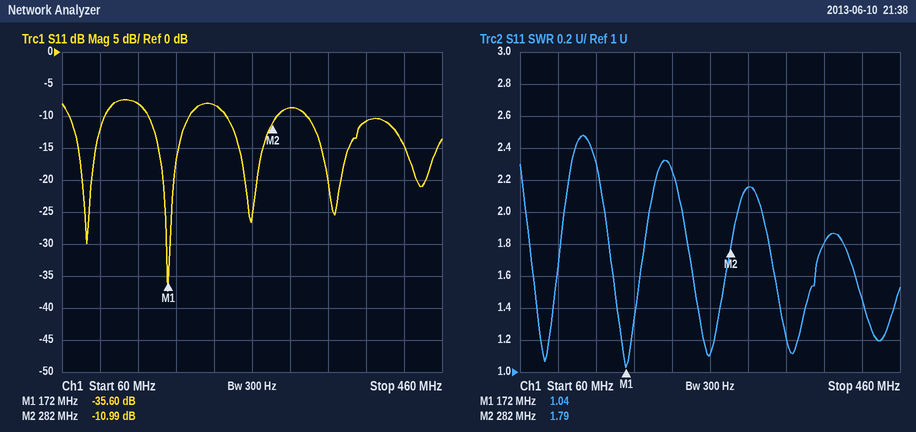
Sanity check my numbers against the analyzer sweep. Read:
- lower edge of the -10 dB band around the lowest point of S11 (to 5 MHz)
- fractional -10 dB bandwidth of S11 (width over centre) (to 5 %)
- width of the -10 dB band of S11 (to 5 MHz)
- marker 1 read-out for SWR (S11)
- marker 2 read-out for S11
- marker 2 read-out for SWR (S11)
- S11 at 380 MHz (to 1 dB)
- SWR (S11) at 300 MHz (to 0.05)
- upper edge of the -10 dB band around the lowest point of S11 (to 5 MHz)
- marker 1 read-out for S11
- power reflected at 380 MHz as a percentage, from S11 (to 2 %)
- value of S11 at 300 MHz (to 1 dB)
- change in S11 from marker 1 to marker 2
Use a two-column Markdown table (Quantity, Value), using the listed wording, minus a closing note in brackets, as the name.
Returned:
| Quantity | Value |
|---|---|
| lower edge of the -10 dB band around the lowest point of S11 | 150 MHz |
| fractional -10 dB bandwidth of S11 (width over centre) | 25 % |
| width of the -10 dB band of S11 | 45 MHz |
| marker 1 read-out for SWR | 1.04 |
| marker 2 read-out for S11 | -10.99 dB |
| marker 2 read-out for SWR | 1.79 |
| S11 at 380 MHz | -11 dB |
| SWR (S11) at 300 MHz | 2.15 |
| upper edge of the -10 dB band around the lowest point of S11 | 195 MHz |
| marker 1 read-out for S11 | -35.60 dB |
| power reflected at 380 MHz as a percentage, from S11 | 8 % |
| value of S11 at 300 MHz | -9 dB |
| change in S11 from marker 1 to marker 2 | 24.61 dB |
